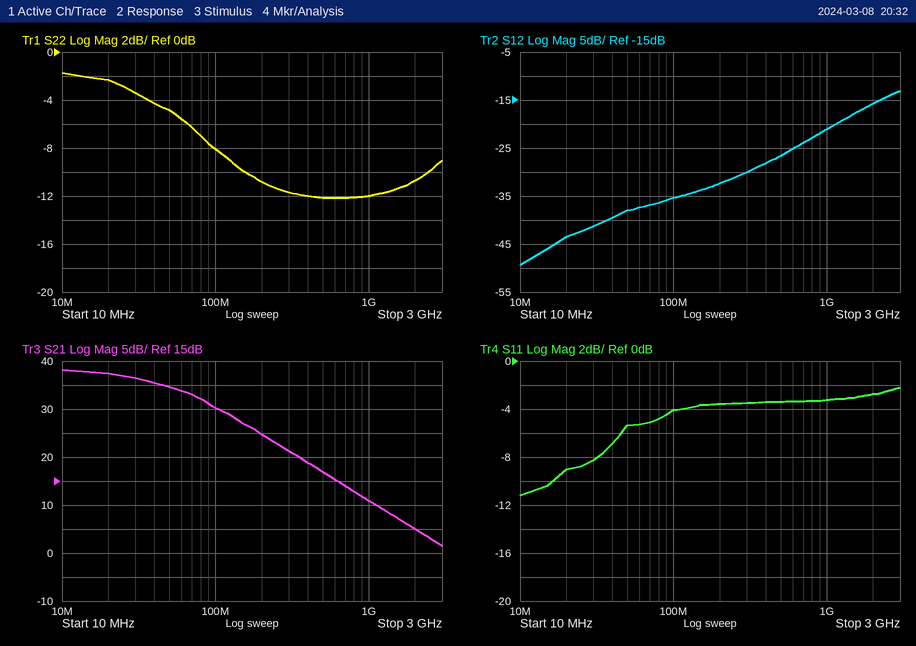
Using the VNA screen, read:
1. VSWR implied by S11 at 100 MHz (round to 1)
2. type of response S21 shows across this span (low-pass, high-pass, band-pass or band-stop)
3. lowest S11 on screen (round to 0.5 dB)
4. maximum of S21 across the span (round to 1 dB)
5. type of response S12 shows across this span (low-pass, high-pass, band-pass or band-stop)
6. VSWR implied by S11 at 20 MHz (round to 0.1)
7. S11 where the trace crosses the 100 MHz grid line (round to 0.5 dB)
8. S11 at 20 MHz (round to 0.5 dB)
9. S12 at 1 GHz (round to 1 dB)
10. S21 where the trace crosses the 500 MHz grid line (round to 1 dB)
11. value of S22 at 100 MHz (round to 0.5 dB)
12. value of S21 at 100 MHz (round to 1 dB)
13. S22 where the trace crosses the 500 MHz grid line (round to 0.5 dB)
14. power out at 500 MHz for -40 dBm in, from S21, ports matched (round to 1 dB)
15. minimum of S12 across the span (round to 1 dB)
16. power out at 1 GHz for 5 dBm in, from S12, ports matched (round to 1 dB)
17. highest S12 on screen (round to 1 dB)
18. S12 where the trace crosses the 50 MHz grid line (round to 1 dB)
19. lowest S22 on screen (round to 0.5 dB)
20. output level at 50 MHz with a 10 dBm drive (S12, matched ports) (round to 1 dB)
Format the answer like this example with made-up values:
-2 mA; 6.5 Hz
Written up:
4; low-pass; -11.0 dB; 38 dB; high-pass; 2.1; -4.0 dB; -9.0 dB; -21 dB; 17 dB; -8.0 dB; 30 dB; -12.0 dB; -23 dBm; -49 dB; -16 dBm; -13 dB; -38 dB; -12.0 dB; -28 dBm
